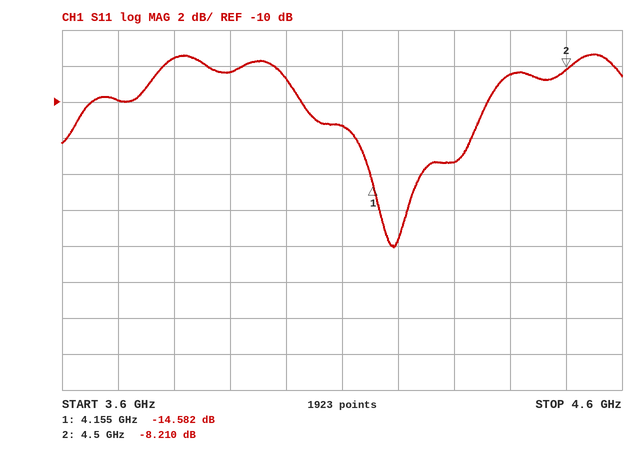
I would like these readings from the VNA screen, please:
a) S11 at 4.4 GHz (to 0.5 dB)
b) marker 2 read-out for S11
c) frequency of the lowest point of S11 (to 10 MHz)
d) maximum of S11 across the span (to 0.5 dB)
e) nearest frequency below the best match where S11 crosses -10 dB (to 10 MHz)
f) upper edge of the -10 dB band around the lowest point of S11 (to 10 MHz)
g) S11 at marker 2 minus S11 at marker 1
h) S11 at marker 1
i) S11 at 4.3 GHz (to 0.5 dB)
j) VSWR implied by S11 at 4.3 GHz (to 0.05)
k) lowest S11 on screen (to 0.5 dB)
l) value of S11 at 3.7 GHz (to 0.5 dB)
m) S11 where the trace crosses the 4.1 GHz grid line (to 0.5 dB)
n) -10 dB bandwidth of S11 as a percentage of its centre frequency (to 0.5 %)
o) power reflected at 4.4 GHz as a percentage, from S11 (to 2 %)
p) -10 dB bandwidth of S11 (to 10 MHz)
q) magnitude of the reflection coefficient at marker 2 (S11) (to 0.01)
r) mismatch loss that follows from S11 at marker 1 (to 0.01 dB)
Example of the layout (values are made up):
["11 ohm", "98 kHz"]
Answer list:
["-8.5 dB", "-8.210 dB", "4.19 GHz", "-7.5 dB", "4.03 GHz", "4.36 GHz", "6.372 dB", "-14.582 dB", "-13.5 dB", "1.55", "-18.0 dB", "-10.0 dB", "-11.5 dB", "8.0 %", "14 %", "330 MHz", "0.39", "0.15 dB"]
